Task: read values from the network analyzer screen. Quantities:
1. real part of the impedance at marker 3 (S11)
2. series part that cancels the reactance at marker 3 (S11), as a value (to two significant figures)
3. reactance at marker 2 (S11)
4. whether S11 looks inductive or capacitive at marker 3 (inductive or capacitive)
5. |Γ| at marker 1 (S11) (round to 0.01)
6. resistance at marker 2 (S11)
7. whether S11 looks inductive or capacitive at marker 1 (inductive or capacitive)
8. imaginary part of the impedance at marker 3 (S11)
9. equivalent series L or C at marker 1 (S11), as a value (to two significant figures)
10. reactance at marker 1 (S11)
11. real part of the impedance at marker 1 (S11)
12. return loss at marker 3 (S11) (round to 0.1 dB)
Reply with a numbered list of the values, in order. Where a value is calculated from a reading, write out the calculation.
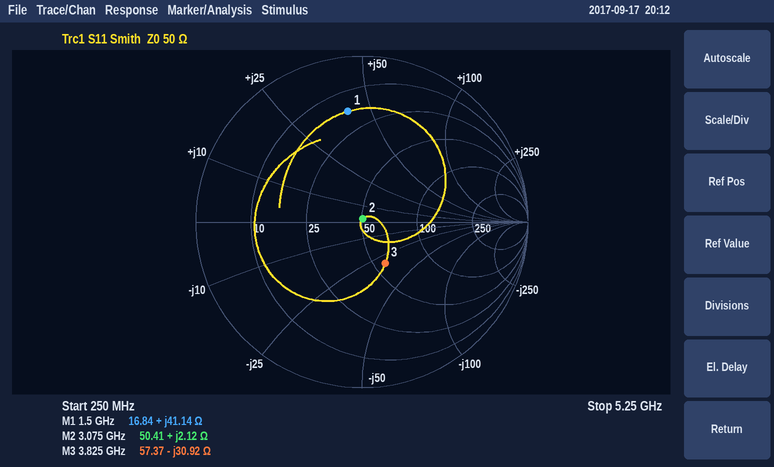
1. 57.37 Ω
2. L = 30.92 Ω/(2π × 3.825 GHz) ≈ 1.3 nH
3. +2.12 Ω
4. capacitive
5. 0.67
6. 50.41 Ω
7. inductive
8. -30.92 Ω
9. L = 41.14 Ω/(2π × 1.5 GHz) ≈ 4.4 nH
10. +41.14 Ω
11. 16.84 Ω
12. 10.9 dB
